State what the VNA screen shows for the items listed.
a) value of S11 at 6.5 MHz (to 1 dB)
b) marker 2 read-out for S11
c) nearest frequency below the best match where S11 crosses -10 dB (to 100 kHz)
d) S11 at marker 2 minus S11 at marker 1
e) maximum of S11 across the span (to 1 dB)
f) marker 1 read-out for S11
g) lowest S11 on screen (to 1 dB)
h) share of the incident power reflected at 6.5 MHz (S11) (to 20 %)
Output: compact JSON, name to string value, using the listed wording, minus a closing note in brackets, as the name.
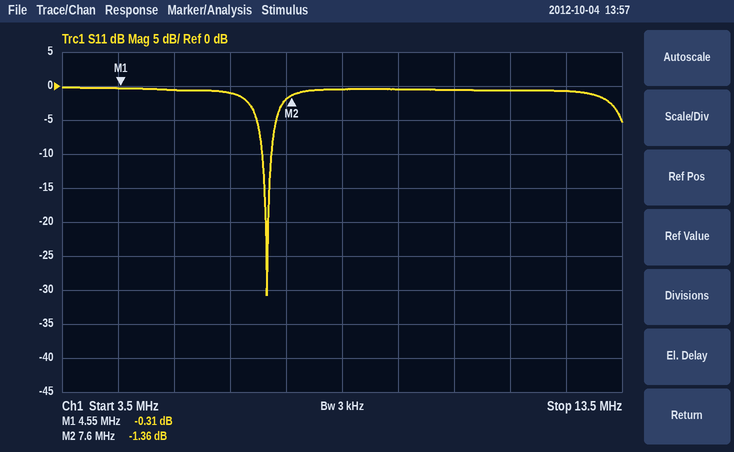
{"value of S11 at 6.5 MHz": "-1 dB", "marker 2 read-out for S11": "-1.36 dB", "nearest frequency below the best match where S11 crosses -10 dB": "7.1 MHz", "S11 at marker 2 minus S11 at marker 1": "-1.05 dB", "maximum of S11 across the span": "0 dB", "marker 1 read-out for S11": "-0.31 dB", "lowest S11 on screen": "-31 dB", "share of the incident power reflected at 6.5 MHz (S11)": "80 %"}
